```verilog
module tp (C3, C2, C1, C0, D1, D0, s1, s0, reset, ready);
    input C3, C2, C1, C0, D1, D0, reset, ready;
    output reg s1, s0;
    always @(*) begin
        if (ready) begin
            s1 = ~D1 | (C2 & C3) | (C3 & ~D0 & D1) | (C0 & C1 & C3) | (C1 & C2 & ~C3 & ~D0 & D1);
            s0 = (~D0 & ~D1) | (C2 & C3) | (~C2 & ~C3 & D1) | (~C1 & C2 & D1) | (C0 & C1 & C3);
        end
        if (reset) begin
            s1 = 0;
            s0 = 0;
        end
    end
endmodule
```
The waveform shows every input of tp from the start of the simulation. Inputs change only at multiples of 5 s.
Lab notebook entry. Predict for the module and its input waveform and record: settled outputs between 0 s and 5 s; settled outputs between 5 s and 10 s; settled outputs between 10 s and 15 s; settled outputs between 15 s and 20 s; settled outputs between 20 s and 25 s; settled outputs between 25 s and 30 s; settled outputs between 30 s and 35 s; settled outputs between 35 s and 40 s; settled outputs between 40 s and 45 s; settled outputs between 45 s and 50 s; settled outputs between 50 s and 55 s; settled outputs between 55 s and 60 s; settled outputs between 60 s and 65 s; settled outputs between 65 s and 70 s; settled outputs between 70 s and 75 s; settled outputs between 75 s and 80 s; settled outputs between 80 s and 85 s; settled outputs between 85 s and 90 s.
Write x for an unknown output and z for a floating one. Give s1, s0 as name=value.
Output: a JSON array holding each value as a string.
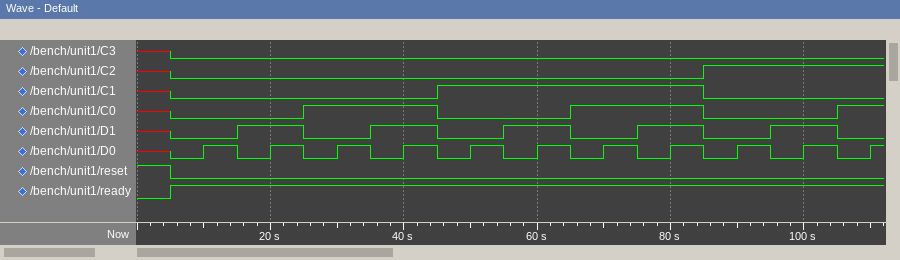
["s1=0, s0=0", "s1=1, s0=1", "s1=1, s0=0", "s1=0, s0=1", "s1=0, s0=1", "s1=1, s0=1", "s1=1, s0=0", "s1=0, s0=1", "s1=0, s0=1", "s1=1, s0=1", "s1=1, s0=0", "s1=0, s0=1", "s1=0, s0=1", "s1=1, s0=1", "s1=1, s0=0", "s1=0, s0=1", "s1=0, s0=1", "s1=1, s0=1"]
